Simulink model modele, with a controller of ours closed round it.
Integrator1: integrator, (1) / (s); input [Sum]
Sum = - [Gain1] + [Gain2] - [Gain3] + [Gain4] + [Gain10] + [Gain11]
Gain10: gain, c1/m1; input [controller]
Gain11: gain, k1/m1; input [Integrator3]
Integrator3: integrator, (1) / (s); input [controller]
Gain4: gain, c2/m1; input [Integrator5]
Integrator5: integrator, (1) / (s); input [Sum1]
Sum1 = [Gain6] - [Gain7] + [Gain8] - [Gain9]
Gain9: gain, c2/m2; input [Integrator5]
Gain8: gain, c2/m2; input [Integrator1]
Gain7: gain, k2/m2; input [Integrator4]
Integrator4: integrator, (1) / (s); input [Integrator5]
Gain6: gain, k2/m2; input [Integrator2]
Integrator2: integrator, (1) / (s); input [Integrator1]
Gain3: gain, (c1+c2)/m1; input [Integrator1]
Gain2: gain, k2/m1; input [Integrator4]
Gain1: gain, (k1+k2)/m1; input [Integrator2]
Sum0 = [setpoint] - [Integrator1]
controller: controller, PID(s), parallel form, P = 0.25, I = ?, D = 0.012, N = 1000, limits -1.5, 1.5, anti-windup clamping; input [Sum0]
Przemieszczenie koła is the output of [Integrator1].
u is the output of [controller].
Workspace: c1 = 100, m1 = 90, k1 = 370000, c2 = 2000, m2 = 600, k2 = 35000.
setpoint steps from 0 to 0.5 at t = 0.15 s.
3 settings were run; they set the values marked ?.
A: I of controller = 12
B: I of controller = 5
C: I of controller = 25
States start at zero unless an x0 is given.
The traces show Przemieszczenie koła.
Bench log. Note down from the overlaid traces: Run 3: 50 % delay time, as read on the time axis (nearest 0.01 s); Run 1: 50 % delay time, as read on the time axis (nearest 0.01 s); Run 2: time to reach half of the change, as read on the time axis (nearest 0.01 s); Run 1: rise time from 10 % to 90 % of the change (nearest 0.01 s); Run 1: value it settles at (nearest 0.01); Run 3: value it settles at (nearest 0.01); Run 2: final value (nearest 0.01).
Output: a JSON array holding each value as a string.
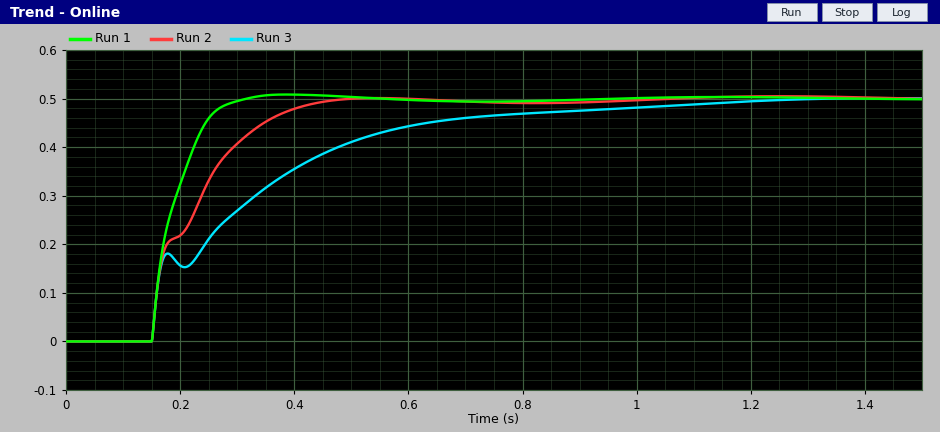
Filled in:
["0.28 s", "0.18 s", "0.22 s", "0.09 s", "0.50", "0.50", "0.50"]
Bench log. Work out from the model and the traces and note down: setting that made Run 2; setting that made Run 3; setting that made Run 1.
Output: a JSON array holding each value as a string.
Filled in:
["A", "B", "C"]
